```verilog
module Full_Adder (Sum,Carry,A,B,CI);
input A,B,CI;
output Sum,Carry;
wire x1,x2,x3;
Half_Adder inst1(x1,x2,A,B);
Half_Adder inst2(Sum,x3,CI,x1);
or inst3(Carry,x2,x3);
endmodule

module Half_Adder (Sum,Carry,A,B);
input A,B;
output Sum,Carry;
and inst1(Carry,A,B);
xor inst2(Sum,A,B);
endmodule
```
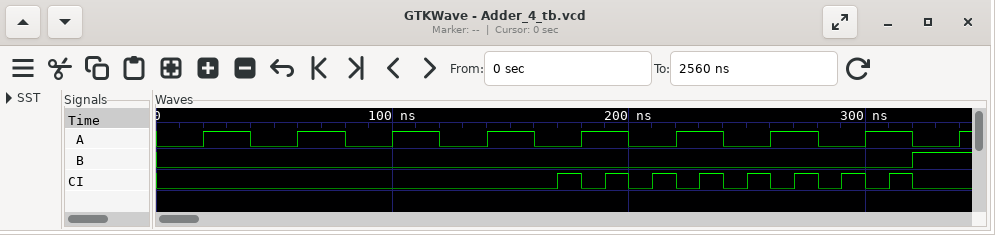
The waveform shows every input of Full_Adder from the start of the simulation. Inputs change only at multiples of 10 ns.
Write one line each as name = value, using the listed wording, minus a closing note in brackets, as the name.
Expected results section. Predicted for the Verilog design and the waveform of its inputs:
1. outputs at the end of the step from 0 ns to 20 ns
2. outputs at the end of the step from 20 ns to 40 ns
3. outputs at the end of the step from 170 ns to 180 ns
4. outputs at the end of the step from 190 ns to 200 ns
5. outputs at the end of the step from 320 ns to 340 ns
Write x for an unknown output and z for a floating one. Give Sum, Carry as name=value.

outputs at the end of the step from 0 ns to 20 ns = Sum=0, Carry=0
outputs at the end of the step from 20 ns to 40 ns = Sum=1, Carry=0
outputs at the end of the step from 170 ns to 180 ns = Sum=1, Carry=0
outputs at the end of the step from 190 ns to 200 ns = Sum=0, Carry=1
outputs at the end of the step from 320 ns to 340 ns = Sum=1, Carry=0
